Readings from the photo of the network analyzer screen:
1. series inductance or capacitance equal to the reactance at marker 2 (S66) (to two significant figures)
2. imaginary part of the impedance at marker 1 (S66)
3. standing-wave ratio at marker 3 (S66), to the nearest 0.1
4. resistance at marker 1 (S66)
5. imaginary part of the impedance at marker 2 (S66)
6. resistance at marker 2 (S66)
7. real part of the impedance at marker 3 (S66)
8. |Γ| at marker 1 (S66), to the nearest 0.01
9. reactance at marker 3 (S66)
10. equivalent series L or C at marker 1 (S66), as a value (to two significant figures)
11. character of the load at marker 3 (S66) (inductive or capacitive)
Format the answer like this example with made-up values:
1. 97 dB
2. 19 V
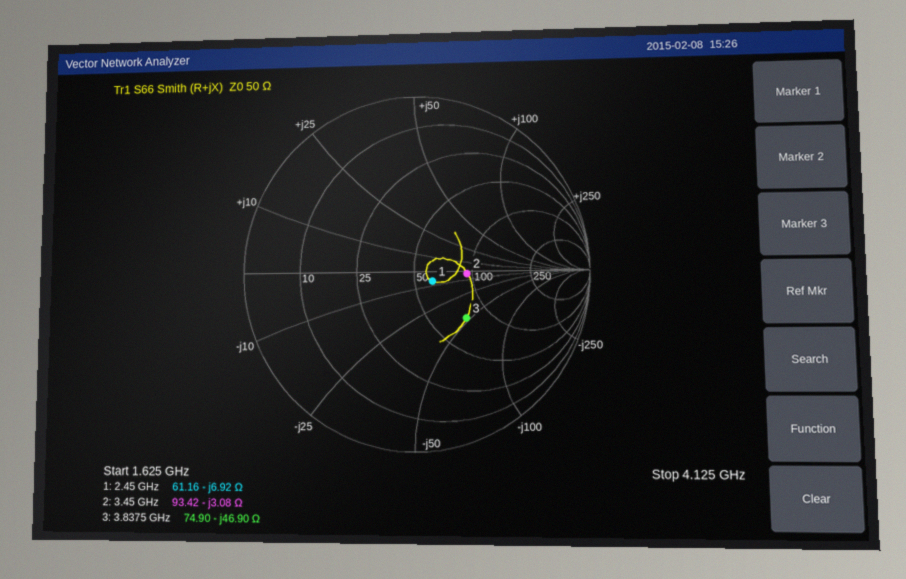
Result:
1. 15 pF
2. -6.92 Ω
3. 2.3
4. 61.16 Ω
5. -3.08 Ω
6. 93.42 Ω
7. 74.90 Ω
8. 0.12
9. -46.90 Ω
10. 9.4 pF
11. capacitive
